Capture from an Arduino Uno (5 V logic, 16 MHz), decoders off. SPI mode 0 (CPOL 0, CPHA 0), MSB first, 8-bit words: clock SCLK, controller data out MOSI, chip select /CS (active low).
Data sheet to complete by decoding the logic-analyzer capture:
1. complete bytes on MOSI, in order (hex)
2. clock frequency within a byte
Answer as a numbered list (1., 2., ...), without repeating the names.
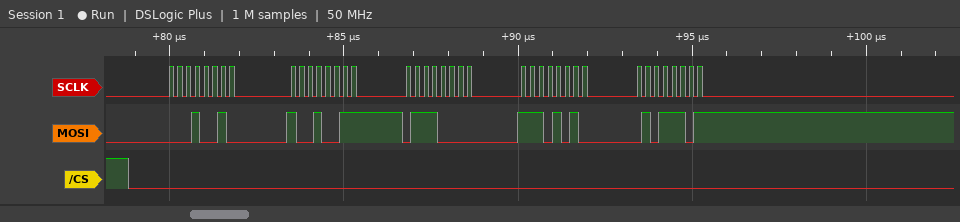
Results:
1. 12 93 70 EA 5D
2. 4 MHz
